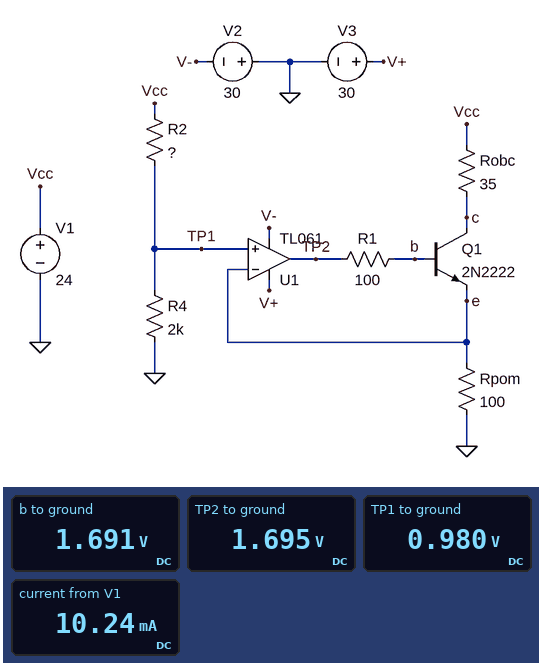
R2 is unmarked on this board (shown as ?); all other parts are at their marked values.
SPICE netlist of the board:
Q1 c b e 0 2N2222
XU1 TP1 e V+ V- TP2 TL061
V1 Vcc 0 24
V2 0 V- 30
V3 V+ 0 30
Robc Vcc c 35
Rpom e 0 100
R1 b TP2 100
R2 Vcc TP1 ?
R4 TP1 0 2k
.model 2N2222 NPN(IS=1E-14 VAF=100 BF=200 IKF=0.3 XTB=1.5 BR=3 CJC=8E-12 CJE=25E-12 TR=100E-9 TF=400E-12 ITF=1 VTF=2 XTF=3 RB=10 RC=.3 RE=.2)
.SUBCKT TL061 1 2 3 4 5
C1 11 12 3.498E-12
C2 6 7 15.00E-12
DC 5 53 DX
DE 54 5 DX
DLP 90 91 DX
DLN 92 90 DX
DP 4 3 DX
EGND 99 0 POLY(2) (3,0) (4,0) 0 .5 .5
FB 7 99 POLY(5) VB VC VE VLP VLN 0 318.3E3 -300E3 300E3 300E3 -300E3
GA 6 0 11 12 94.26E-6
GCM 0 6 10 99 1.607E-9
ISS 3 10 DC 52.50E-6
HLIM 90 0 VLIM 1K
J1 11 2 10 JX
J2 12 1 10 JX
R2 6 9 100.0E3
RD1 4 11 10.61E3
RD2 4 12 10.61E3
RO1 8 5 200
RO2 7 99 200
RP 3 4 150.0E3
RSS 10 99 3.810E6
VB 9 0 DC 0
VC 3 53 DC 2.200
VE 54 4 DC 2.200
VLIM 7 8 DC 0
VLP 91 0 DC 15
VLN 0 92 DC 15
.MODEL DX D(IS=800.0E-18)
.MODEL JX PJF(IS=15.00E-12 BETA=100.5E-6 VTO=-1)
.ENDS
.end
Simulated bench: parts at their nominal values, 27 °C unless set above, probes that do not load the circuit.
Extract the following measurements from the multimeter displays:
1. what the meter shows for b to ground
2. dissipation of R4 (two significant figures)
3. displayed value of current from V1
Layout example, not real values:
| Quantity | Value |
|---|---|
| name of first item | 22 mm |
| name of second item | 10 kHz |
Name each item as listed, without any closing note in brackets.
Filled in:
| Quantity | Value |
|---|---|
| what the meter shows for b to ground | 1.691 V |
| dissipation of R4 | 480 µW |
| displayed value of current from V1 | 10.24 mA |
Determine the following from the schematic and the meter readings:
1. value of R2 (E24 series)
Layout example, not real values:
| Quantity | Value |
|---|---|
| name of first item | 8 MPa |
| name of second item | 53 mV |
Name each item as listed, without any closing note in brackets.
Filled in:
| Quantity | Value |
|---|---|
| value of R2 | 47 kΩ |
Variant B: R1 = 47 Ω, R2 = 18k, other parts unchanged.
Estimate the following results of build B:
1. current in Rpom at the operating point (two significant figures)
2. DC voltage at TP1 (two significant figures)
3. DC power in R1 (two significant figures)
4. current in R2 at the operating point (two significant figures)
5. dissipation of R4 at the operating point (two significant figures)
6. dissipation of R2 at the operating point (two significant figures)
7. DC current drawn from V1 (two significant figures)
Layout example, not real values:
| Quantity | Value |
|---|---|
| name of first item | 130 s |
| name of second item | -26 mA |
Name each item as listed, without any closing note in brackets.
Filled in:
| Quantity | Value |
|---|---|
| current in Rpom at the operating point | 24 mA |
| DC voltage at TP1 | 2.4 V |
| DC power in R1 | 530 nW |
| current in R2 at the operating point | 1.2 mA |
| dissipation of R4 at the operating point | 2.9 mW |
| dissipation of R2 at the operating point | 26 mW |
| DC current drawn from V1 | 25 mA |
